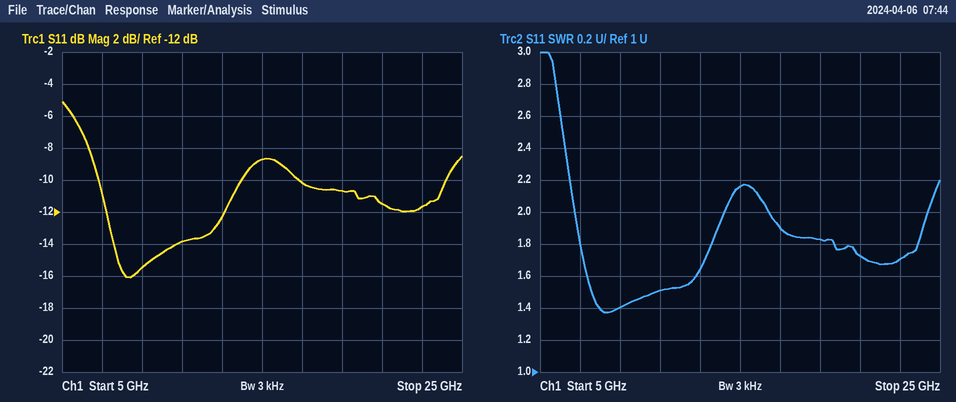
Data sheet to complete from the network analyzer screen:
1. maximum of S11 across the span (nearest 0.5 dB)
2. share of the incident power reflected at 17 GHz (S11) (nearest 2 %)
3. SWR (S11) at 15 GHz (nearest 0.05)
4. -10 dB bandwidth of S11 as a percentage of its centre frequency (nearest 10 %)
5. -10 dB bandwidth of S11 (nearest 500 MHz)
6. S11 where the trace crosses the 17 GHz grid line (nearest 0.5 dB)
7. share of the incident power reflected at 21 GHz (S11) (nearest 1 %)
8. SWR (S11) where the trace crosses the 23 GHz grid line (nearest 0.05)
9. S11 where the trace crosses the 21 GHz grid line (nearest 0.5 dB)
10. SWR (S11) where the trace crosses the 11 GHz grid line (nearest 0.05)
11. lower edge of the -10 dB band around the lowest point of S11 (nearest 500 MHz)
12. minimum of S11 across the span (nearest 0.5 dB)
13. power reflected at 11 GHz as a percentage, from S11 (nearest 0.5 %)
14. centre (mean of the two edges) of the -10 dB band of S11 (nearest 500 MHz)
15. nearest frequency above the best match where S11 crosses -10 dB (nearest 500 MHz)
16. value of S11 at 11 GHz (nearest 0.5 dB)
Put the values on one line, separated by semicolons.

-5.0 dB; 10 %; 2.15; 70 %; 7.0 GHz; -10.0 dB; 7 %; 1.70; -11.5 dB; 1.50; 7.0 GHz; -16.0 dB; 4.0 %; 10.5 GHz; 14.0 GHz; -14.0 dB
